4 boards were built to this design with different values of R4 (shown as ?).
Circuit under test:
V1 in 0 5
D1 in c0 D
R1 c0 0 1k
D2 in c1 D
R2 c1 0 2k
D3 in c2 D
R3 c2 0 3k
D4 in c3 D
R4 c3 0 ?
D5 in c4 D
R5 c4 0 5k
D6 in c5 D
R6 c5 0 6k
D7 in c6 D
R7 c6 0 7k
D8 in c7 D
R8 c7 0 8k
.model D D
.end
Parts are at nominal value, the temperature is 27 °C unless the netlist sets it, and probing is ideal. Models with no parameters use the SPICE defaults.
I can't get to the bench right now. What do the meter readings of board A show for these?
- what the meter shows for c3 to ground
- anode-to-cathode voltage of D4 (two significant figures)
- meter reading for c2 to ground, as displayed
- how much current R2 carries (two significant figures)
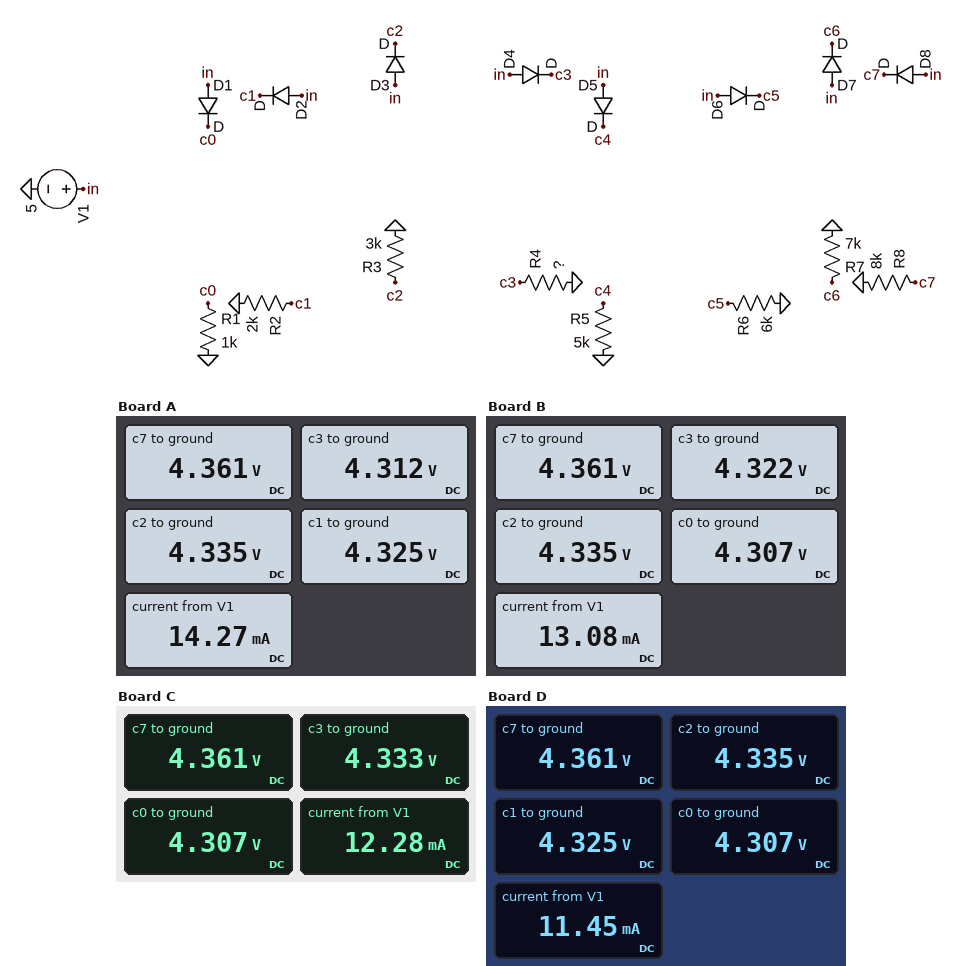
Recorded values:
4.312 V
690 mV
4.335 V
2.2 mA
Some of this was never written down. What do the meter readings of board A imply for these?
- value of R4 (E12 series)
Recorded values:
1.2 kΩ
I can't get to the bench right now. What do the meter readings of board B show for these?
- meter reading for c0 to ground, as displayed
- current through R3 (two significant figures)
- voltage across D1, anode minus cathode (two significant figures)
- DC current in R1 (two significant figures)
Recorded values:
4.307 V
1.4 mA
690 mV
4.3 mA
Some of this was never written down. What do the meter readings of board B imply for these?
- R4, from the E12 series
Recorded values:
1.8 kΩ
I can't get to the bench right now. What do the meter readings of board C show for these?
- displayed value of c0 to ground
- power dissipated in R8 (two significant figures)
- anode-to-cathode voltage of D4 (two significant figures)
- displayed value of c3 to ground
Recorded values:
4.307 V
2.4 mW
670 mV
4.333 V
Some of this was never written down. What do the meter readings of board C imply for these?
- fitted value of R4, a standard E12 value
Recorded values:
2.7 kΩ
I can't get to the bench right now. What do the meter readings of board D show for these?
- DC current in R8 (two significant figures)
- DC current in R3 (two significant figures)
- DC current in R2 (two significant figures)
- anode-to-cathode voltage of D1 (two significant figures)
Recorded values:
550 µA
1.4 mA
2.2 mA
690 mV
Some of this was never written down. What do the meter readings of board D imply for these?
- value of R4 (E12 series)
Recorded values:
5.6 kΩ
